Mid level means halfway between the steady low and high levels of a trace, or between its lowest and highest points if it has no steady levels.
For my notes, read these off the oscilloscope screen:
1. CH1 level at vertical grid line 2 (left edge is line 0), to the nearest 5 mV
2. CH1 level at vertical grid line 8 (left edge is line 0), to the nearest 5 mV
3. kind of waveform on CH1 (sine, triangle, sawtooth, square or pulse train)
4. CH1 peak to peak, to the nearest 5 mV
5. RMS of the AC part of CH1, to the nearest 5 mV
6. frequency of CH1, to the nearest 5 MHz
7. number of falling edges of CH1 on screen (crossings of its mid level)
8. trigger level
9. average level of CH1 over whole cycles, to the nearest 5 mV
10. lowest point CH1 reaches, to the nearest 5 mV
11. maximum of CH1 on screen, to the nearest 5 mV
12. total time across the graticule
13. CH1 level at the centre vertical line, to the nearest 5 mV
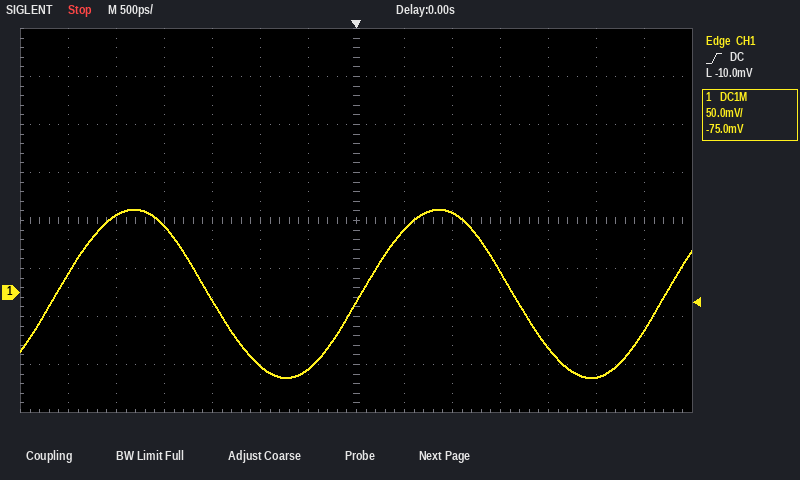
80 mV
65 mV
sine
175 mV
60 mV
315 MHz
2
-10.0 mV
0 mV
-90 mV
85 mV
7 ns
-10 mV
